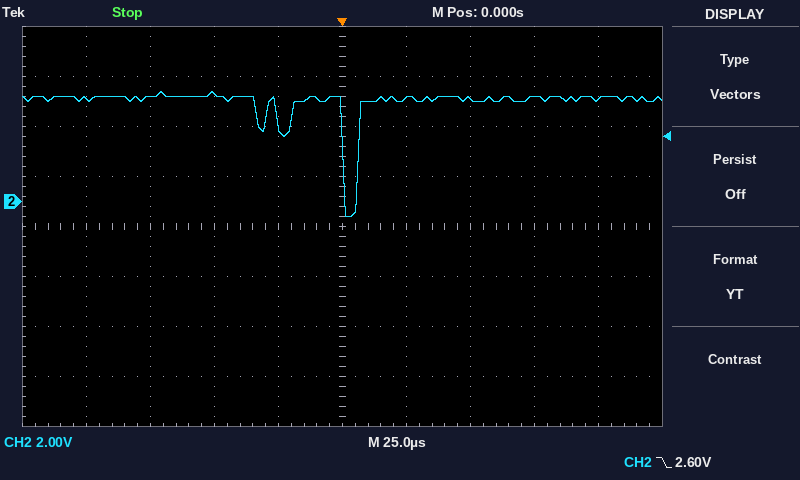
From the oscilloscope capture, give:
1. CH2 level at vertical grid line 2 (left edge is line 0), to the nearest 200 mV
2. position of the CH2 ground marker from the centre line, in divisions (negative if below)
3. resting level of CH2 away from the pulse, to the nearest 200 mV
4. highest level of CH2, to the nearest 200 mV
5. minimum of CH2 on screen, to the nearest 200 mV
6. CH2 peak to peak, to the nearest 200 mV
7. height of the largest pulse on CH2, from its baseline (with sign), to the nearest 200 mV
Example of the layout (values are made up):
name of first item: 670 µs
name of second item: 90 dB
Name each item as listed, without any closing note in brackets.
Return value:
CH2 level at vertical grid line 2 (left edge is line 0), to the nearest 200 mV: 4.2 V
position of the CH2 ground marker from the centre line, in divisions: +0.5 div
resting level of CH2 away from the pulse, to the nearest 200 mV: 4.2 V
highest level of CH2, to the nearest 200 mV: 4.4 V
minimum of CH2 on screen, to the nearest 200 mV: -600 mV
CH2 peak to peak, to the nearest 200 mV: 5.0 V
height of the largest pulse on CH2, from its baseline (with sign), to the nearest 200 mV: -4.8 V
